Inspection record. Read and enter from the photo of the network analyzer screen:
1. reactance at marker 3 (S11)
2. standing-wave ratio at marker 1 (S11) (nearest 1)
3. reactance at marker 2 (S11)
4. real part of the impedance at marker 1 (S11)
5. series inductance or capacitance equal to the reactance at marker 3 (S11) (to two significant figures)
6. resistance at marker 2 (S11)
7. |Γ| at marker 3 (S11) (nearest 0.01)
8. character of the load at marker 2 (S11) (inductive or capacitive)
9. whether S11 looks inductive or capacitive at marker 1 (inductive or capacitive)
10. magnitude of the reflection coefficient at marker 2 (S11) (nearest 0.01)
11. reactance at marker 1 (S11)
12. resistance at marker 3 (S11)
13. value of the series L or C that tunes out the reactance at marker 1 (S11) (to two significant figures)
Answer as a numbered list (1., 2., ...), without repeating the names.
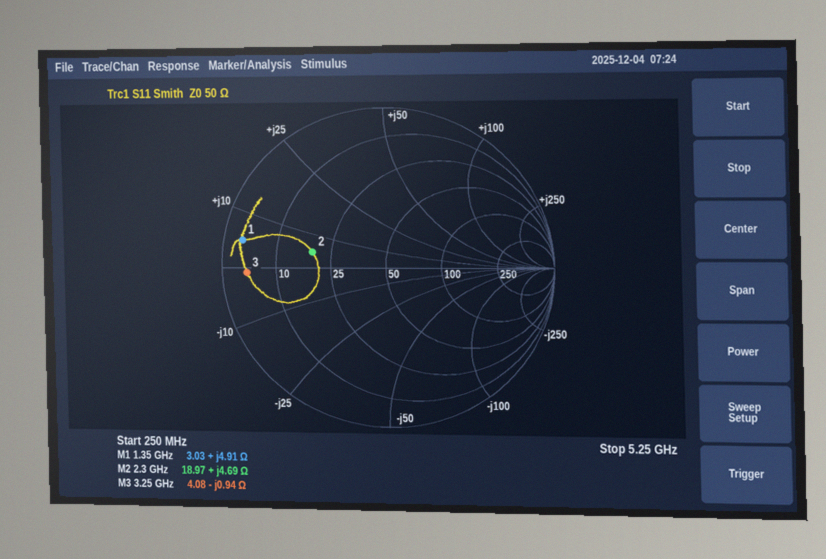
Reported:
1. -0.94 Ω
2. 17
3. +4.69 Ω
4. 3.03 Ω
5. 52 pF
6. 18.97 Ω
7. 0.85
8. inductive
9. inductive
10. 0.45
11. +4.91 Ω
12. 4.08 Ω
13. 24 pF
